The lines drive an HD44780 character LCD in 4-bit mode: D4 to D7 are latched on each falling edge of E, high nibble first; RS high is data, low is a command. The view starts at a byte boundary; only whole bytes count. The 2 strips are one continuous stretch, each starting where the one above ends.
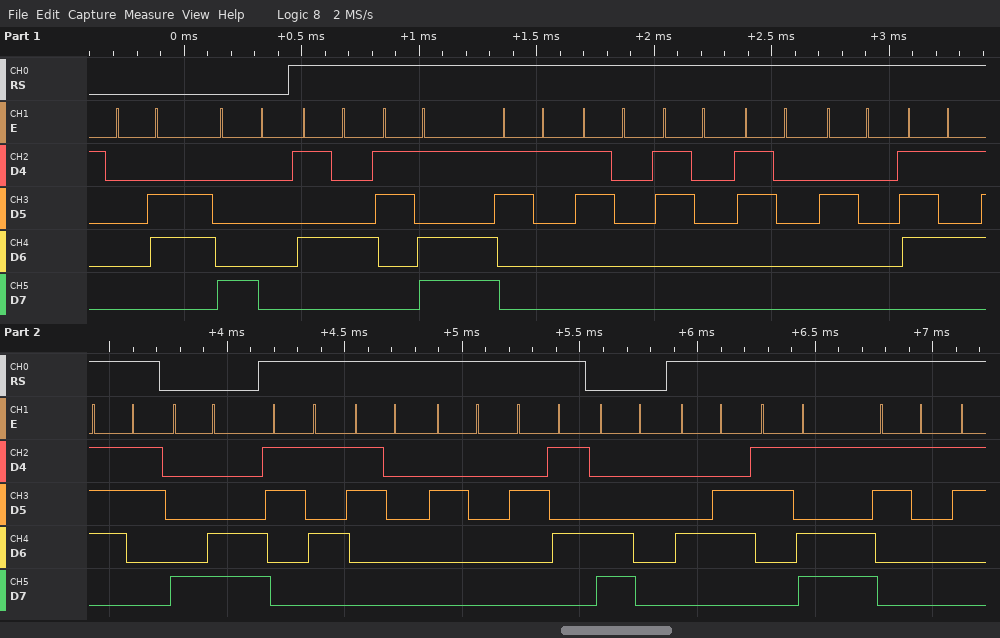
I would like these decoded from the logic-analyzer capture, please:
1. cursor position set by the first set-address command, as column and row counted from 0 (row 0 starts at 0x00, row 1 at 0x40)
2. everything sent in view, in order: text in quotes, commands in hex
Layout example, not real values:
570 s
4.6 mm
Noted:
column 0, row 0
0x06 0x80 "T=1000 us" 0x8C "50 %" 0xC0 "F=1"
